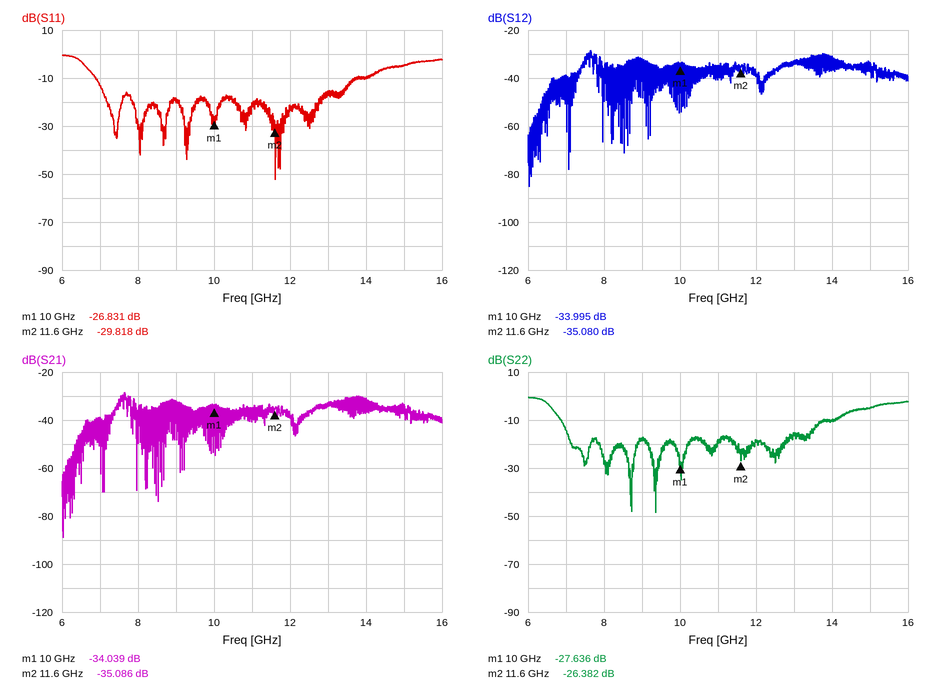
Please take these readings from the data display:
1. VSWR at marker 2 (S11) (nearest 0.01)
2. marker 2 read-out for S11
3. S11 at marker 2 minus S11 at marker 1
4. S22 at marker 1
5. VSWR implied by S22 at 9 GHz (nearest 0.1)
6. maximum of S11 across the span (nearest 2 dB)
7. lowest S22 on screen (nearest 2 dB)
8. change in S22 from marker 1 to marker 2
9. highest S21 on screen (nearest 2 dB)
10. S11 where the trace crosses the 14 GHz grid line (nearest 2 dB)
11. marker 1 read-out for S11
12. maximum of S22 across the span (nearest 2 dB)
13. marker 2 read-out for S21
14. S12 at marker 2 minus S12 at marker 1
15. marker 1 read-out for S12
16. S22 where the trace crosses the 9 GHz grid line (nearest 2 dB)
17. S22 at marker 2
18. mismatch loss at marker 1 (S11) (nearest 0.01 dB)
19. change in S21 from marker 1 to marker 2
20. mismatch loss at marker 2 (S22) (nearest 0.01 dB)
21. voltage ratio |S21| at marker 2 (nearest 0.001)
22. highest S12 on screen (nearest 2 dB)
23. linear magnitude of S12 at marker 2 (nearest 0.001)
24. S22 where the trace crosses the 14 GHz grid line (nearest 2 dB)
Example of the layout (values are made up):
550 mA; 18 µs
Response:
1.07; -29.818 dB; -2.987 dB; -27.636 dB; 1.3; 0 dB; -48 dB; 1.254 dB; -28 dB; -10 dB; -26.831 dB; 0 dB; -35.086 dB; -1.085 dB; -33.995 dB; -18 dB; -26.382 dB; 0.01 dB; -1.047 dB; 0.01 dB; 0.018; -28 dB; 0.018; -10 dB
